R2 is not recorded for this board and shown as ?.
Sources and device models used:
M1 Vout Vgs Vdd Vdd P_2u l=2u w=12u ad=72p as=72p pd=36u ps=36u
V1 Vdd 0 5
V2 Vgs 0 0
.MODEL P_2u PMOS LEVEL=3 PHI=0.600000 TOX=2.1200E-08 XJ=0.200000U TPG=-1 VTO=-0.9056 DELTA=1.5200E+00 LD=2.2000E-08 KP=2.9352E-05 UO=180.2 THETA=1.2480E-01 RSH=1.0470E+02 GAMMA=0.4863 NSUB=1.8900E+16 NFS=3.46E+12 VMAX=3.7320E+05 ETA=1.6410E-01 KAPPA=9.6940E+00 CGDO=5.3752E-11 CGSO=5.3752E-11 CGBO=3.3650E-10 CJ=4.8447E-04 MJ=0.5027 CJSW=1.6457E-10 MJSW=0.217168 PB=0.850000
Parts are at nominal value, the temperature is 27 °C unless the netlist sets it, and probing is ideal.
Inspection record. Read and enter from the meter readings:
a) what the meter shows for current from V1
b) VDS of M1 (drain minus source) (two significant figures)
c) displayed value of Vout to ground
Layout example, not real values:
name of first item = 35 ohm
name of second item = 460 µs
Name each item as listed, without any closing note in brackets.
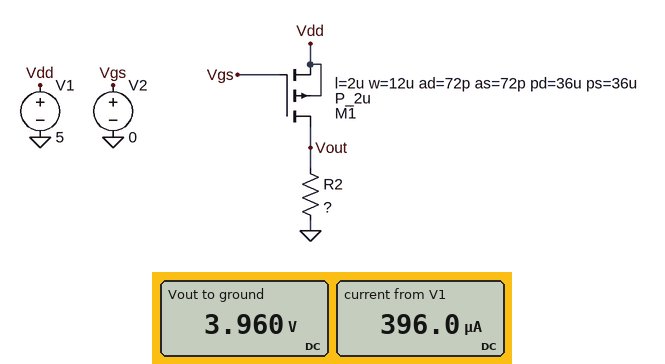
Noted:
what the meter shows for current from V1 = 396.0 µA
VDS of M1 (drain minus source) = -1.0 V
displayed value of Vout to ground = 3.960 V
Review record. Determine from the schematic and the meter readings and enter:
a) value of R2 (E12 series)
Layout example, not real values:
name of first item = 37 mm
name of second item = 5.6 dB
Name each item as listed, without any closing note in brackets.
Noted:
value of R2 = 10 kΩ
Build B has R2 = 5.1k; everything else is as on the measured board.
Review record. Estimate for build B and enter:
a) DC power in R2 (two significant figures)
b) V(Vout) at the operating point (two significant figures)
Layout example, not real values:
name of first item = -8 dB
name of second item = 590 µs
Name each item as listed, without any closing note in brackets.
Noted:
DC power in R2 = 1.9 mW
V(Vout) at the operating point = 3.1 V
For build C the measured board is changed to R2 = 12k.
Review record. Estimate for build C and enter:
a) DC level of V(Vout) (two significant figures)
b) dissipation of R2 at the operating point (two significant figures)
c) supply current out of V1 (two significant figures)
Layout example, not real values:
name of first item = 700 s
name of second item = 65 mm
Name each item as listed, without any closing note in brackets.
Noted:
DC level of V(Vout) = 4.1 V
dissipation of R2 at the operating point = 1.4 mW
supply current out of V1 = 340 µA
